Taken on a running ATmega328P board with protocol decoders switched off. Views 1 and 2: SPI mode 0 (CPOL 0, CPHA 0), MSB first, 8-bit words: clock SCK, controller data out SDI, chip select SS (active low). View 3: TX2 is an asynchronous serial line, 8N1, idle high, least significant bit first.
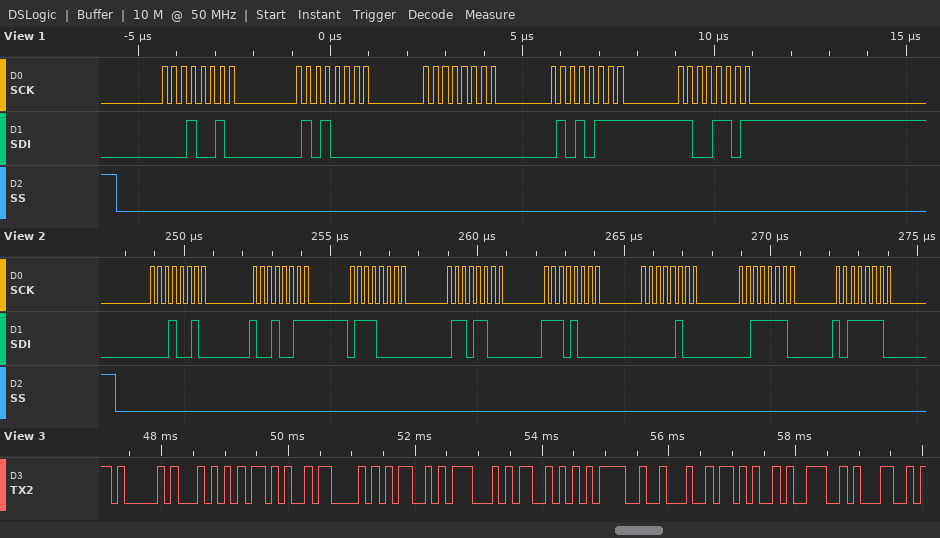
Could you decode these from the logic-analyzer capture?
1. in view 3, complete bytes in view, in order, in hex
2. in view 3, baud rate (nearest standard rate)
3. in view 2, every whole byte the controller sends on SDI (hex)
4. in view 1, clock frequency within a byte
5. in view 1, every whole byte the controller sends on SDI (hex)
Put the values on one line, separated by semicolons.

41 54 2B 43 4D 47 53 3D 22 2B 39 31; 9600 baud; 12 93 70 6C E8 04 3E BE; 4 MHz; 0x12 0x50 0x00 0x57 0xCD
